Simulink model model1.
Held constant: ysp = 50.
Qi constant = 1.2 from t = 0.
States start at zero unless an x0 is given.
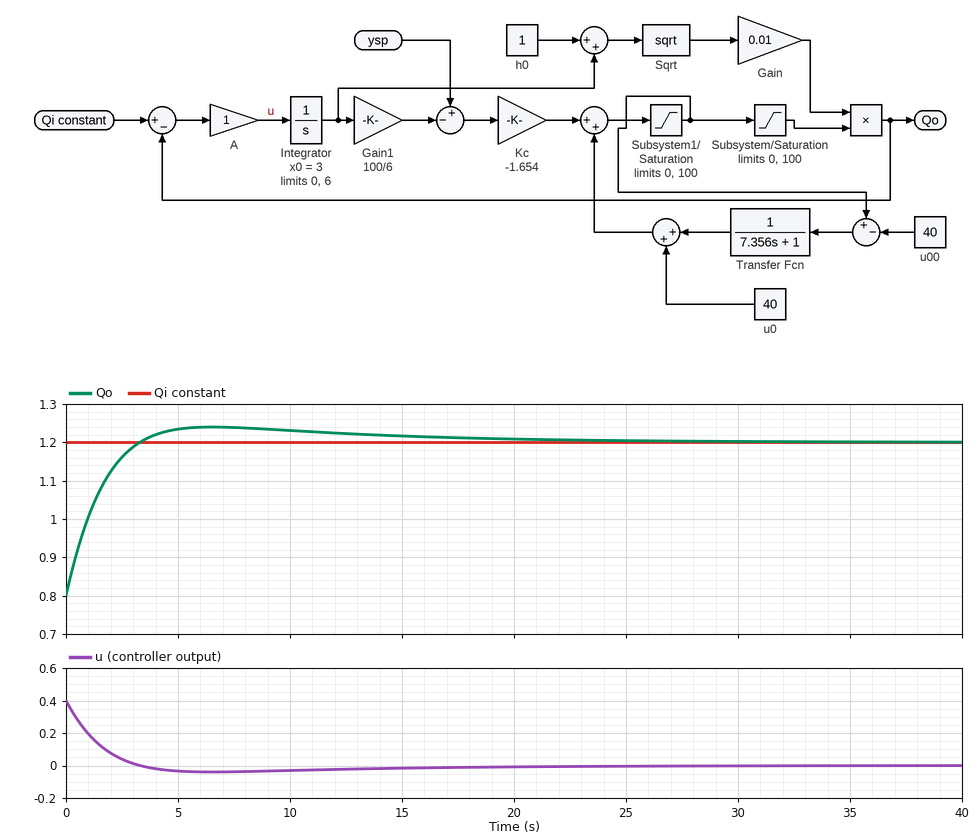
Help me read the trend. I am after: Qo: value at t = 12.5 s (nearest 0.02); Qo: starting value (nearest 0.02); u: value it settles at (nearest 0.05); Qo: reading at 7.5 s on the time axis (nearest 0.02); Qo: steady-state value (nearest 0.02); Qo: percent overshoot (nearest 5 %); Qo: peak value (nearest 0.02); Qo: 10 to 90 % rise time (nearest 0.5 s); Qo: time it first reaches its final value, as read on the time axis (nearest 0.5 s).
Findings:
1.22
0.80
0.00
1.24
1.20
10 %
1.24
2.5 s
3.5 s
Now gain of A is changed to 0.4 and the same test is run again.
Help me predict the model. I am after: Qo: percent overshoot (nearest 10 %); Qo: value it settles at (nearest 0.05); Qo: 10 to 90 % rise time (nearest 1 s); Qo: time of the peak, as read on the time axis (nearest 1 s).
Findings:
20 %
1.20
5 s
12 s
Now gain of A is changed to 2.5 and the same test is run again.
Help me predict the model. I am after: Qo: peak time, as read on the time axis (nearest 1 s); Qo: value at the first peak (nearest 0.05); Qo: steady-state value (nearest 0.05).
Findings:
3 s
1.20
1.20
